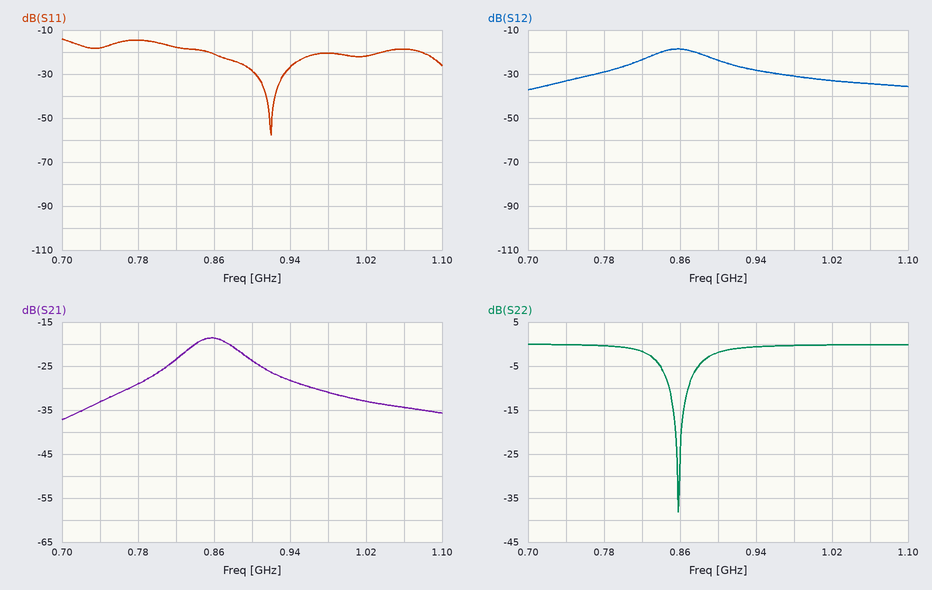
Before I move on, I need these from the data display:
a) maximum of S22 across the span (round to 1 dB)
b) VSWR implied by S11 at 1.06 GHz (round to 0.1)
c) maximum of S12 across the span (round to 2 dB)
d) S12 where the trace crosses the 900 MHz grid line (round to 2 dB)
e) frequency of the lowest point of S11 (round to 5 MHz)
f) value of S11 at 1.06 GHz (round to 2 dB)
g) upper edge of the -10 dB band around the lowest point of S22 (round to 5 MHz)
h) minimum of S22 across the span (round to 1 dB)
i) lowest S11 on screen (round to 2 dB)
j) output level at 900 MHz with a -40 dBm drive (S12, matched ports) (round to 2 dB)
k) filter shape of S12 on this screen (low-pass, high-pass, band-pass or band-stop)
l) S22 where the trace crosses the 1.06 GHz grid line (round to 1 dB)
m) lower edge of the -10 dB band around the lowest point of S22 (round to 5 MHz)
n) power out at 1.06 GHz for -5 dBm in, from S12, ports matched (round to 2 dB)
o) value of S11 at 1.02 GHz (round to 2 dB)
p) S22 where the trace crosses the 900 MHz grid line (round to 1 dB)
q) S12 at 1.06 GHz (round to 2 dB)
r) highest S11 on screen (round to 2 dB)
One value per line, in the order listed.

0 dB
1.3
-18 dB
-24 dB
920 MHz
-18 dB
870 MHz
-38 dB
-58 dB
-64 dBm
band-pass
0 dB
850 MHz
-40 dBm
-22 dB
-2 dB
-34 dB
-14 dB
